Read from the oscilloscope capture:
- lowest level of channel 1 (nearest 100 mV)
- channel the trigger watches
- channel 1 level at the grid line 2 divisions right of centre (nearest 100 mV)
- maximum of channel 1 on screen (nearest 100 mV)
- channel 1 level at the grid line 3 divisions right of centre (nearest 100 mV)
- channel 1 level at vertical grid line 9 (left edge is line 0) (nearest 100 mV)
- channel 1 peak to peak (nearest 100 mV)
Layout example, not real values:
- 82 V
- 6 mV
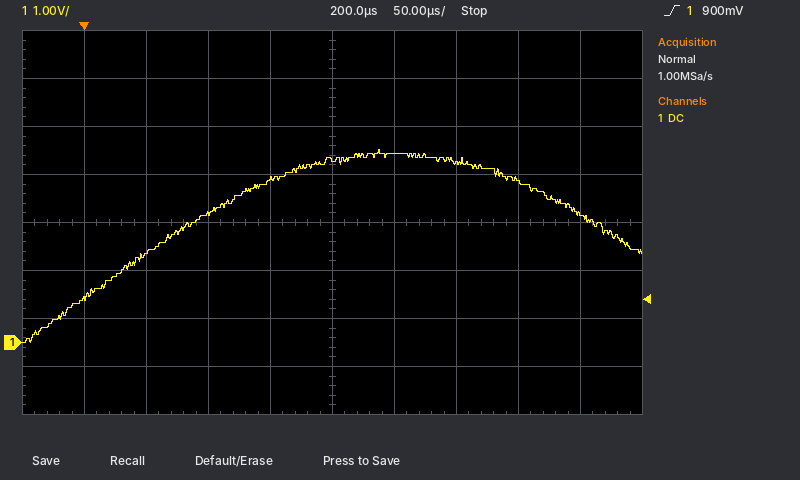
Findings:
- 0.0 V
- channel 1
- 3.7 V
- 4.0 V
- 3.4 V
- 2.7 V
- 4.0 V
